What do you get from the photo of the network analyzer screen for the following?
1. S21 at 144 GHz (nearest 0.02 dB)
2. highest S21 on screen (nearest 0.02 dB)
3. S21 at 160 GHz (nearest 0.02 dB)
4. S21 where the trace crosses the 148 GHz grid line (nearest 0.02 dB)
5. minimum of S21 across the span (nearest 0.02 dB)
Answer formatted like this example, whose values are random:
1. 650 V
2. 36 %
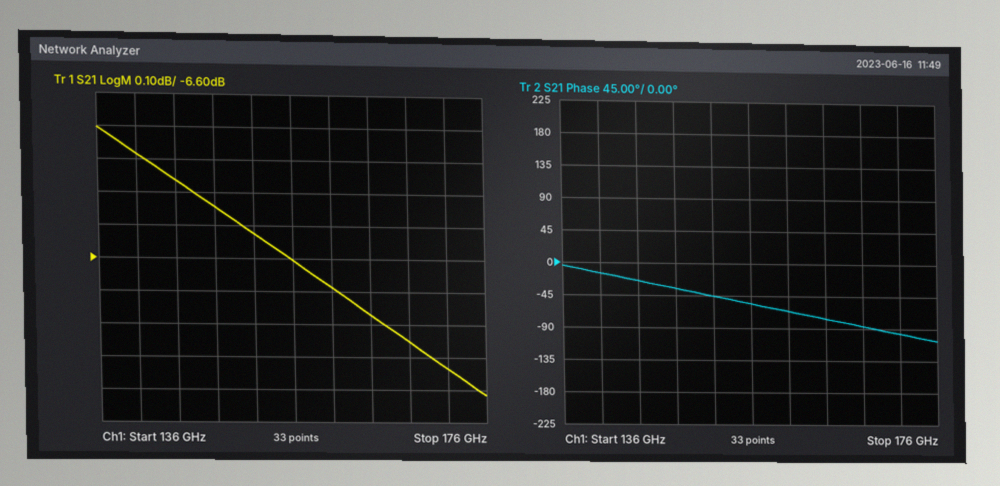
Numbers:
1. -6.36 dB
2. -6.20 dB
3. -6.68 dB
4. -6.44 dB
5. -7.02 dB
